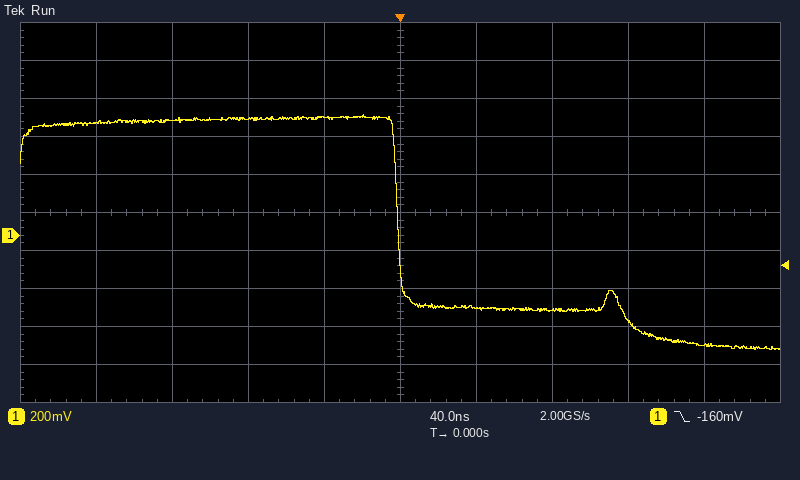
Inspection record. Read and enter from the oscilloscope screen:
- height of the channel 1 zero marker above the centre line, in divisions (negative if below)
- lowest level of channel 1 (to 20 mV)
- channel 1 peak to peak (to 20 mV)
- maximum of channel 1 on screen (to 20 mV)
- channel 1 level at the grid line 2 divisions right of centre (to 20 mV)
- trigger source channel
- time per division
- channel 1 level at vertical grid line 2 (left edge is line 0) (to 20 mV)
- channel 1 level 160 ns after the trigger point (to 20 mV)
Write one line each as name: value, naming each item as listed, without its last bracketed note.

height of the channel 1 zero marker above the centre line, in divisions: -0.6 div
lowest level of channel 1: -600 mV
channel 1 peak to peak: 1.24 V
maximum of channel 1 on screen: 640 mV
channel 1 level at the grid line 2 divisions right of centre: -400 mV
trigger source channel: channel 1
time per division: 40 ns
channel 1 level at vertical grid line 2 (left edge is line 0): 600 mV
channel 1 level 160 ns after the trigger point: -580 mV
